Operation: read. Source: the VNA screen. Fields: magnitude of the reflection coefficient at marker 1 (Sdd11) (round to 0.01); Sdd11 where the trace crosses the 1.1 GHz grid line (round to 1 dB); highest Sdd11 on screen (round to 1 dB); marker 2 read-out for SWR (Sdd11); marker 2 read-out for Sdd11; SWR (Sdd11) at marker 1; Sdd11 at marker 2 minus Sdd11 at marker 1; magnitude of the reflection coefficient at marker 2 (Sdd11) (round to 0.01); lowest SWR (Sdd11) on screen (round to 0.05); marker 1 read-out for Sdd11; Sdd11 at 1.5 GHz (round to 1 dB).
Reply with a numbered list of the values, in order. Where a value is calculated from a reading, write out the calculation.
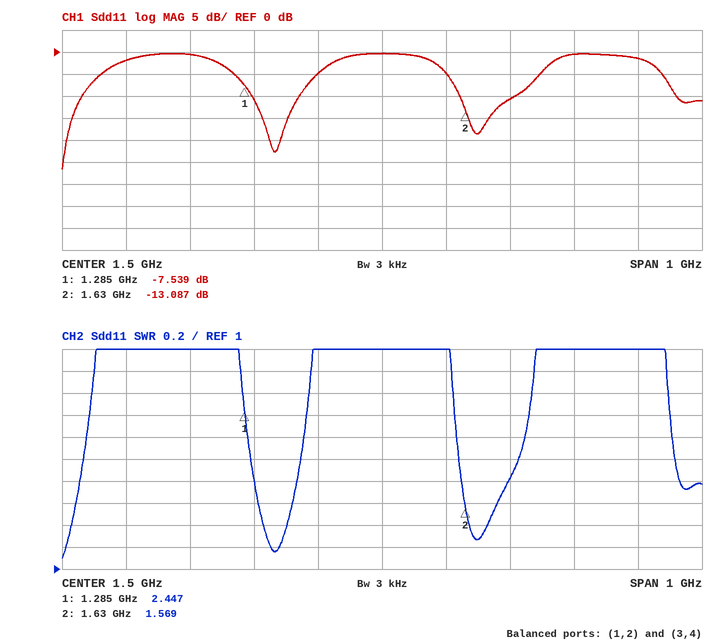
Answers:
1. 10^(-7.539/20) ≈ 0.42
2. -2 dB
3. 0 dB
4. 1.569
5. -13.087 dB
6. 2.447
7. -13.087 − (-7.539) = -5.548 dB
8. 10^(-13.087/20) ≈ 0.22
9. 1.10
10. -7.539 dB
11. 0 dB
